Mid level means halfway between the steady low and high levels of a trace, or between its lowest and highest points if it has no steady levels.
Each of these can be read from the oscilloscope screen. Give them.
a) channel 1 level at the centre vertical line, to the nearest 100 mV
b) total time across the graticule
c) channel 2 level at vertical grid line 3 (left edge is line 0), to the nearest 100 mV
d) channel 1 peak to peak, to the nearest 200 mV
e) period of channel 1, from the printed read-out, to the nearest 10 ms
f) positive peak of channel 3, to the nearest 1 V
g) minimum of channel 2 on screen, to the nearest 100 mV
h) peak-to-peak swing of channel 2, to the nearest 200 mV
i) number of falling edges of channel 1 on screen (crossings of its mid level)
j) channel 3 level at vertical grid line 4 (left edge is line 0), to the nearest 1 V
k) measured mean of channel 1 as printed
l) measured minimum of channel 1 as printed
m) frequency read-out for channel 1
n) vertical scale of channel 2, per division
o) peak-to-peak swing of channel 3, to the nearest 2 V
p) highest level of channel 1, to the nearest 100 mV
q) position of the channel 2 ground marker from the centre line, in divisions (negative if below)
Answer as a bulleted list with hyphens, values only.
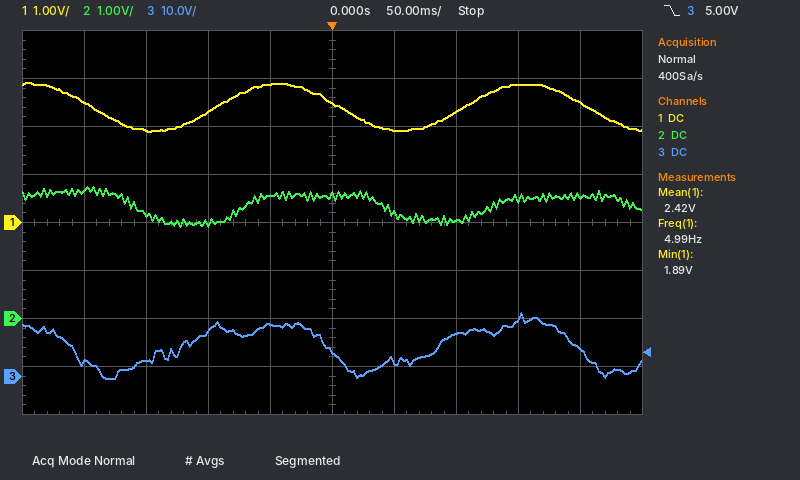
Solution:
- 2.5 V
- 500 ms
- 2.0 V
- 1.0 V
- 200 ms
- 13 V
- 1.9 V
- 800 mV
- 3
- 11 V
- 2.42 V
- 1.89 V
- 4.99 Hz
- 1 V
- 14 V
- 2.9 V
- -2.0 div
